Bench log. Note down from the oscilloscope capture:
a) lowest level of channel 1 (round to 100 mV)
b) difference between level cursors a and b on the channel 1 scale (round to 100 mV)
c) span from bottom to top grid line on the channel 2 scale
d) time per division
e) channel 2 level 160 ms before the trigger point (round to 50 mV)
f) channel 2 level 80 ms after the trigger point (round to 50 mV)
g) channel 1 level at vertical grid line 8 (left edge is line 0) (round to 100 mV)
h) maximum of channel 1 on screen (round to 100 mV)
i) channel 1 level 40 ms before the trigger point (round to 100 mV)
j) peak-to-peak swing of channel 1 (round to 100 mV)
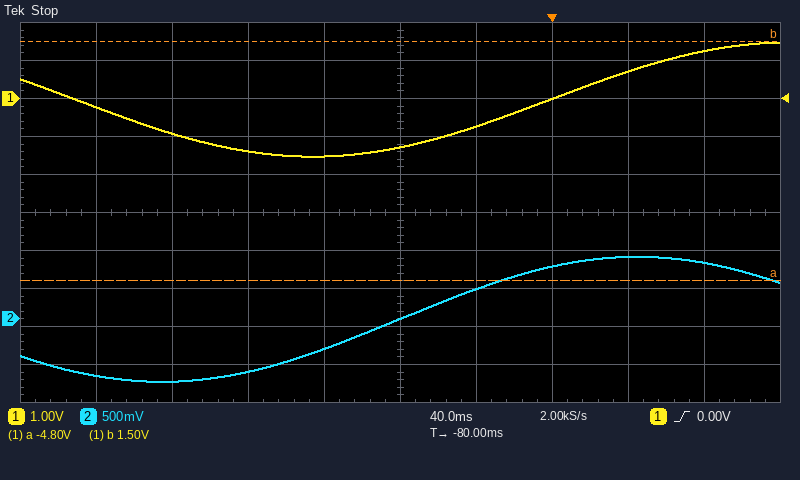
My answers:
-1.5 V
6.3 V
5 V
40 ms
-700 mV
750 mV
700 mV
1.5 V
-700 mV
3.0 V
